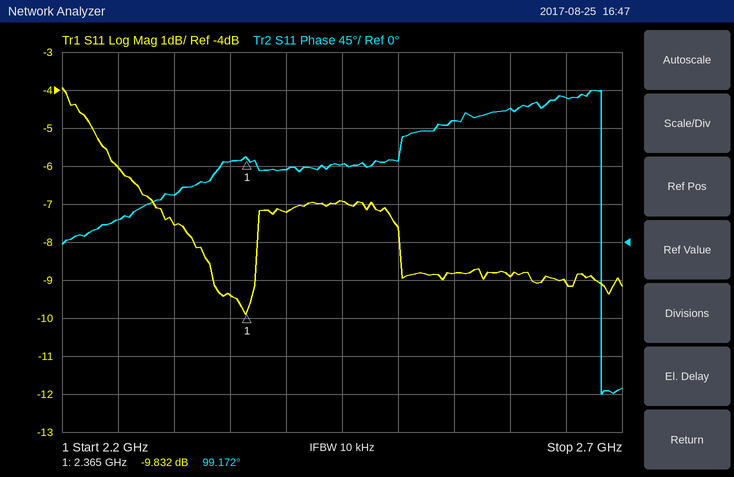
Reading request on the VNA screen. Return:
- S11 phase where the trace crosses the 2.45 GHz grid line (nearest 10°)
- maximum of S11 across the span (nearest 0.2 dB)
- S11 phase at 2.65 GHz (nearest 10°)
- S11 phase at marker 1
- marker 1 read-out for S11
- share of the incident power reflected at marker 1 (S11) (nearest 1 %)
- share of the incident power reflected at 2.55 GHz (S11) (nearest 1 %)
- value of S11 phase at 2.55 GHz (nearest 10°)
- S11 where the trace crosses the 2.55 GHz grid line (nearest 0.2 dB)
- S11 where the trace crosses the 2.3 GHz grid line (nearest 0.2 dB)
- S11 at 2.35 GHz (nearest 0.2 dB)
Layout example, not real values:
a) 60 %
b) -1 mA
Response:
a) 90°
b) -4.0 dB
c) 170°
d) 99.172°
e) -9.832 dB
f) 10 %
g) 13 %
h) 140°
i) -8.8 dB
j) -7.6 dB
k) -9.4 dB
